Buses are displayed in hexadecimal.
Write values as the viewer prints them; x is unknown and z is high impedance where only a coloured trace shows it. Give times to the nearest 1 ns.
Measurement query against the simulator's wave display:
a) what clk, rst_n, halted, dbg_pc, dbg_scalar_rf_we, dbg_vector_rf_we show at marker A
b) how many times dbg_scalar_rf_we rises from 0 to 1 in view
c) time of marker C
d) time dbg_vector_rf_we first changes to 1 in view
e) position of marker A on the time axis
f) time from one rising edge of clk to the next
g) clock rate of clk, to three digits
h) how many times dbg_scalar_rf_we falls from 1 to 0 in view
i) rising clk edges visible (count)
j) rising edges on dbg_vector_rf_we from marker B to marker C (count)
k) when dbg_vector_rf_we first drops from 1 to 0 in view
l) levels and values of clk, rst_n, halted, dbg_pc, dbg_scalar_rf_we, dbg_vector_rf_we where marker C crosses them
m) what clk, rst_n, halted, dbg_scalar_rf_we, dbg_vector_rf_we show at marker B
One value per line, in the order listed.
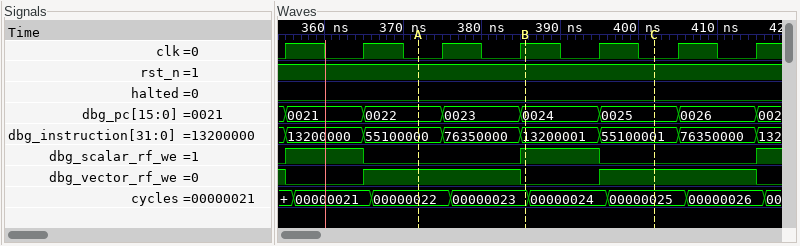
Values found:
clk=0, rst_n=1, halted=0, dbg_pc=0022, dbg_scalar_rf_we=0, dbg_vector_rf_we=1
3
402 ns
365 ns
372 ns
10 ns
100 MHz
2
7
1
355 ns
clk=0, rst_n=1, halted=0, dbg_pc=0025, dbg_scalar_rf_we=0, dbg_vector_rf_we=1
clk=1, rst_n=1, halted=0, dbg_scalar_rf_we=1, dbg_vector_rf_we=0
